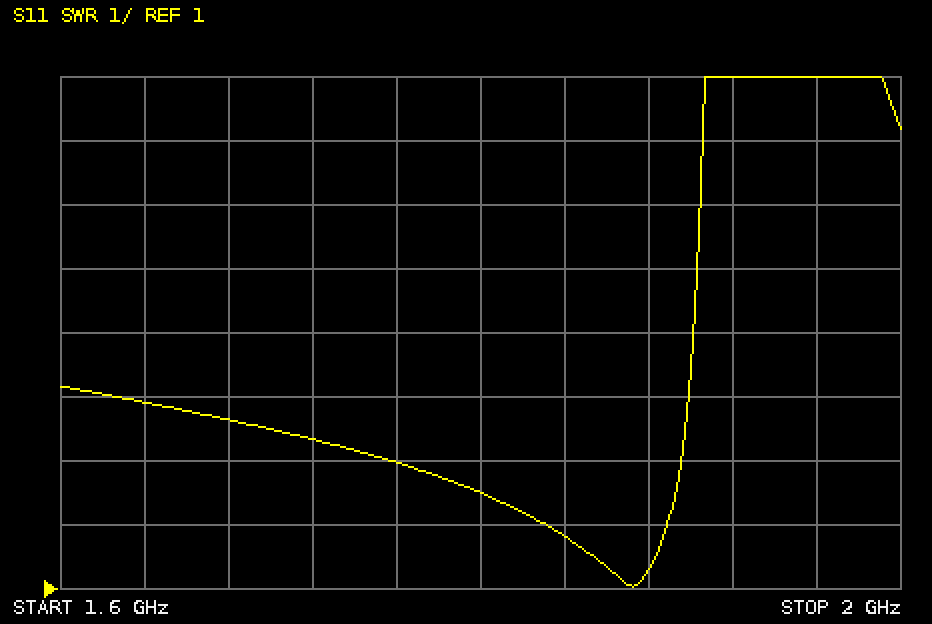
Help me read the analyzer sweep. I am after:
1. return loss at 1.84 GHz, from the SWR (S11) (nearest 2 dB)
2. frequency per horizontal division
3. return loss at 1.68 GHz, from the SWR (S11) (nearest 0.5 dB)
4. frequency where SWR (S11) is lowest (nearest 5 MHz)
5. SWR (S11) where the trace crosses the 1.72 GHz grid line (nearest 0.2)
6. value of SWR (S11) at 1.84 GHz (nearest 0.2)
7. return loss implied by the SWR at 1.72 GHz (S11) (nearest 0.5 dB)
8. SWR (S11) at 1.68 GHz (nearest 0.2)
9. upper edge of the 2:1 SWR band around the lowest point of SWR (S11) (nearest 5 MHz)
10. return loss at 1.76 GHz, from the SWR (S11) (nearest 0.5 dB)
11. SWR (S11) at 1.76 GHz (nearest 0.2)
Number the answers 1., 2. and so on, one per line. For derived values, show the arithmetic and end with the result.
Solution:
1. −20 log10((1.8 − 1)/(1.8 + 1)) ≈ 10.9 dB, so 10 dB to the nearest 2 dB
2. 40 MHz
3. −20 log10((3.6 − 1)/(3.6 + 1)) ≈ 5.0 dB
4. 1.870 GHz
5. 3.4
6. 1.8
7. −20 log10((3.4 − 1)/(3.4 + 1)) ≈ 5.26 dB, so 5.5 dB to the nearest 0.5 dB
8. 3.6
9. 1.890 GHz
10. −20 log10((3 − 1)/(3 + 1)) ≈ 6.0 dB
11. 3.0
